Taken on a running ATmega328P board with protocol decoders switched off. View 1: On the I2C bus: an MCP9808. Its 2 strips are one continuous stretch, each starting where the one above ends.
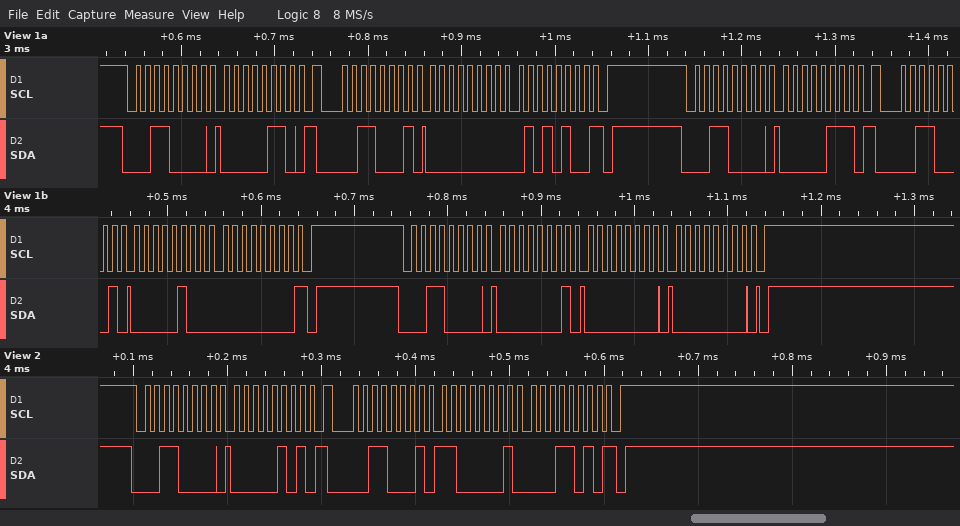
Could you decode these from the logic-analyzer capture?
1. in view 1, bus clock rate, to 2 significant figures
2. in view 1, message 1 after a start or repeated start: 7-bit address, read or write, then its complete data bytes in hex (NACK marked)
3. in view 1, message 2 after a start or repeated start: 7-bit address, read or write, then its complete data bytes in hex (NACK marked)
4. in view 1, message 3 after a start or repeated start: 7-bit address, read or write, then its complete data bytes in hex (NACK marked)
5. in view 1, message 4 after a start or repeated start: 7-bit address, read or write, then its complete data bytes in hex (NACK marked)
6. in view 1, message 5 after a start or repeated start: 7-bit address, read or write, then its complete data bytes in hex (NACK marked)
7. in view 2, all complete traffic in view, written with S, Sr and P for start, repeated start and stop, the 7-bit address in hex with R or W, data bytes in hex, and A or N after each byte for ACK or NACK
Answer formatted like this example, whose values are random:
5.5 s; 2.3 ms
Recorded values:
100 kHz; 0x18 write: 06; 0x18 read: 00 54 NACK; 0x18 write: 07; 0x18 read: 04 00 NACK; 0x18 write: 01 00 00; S 18W A 05 A Sr 18R A C1 A 1A N P
